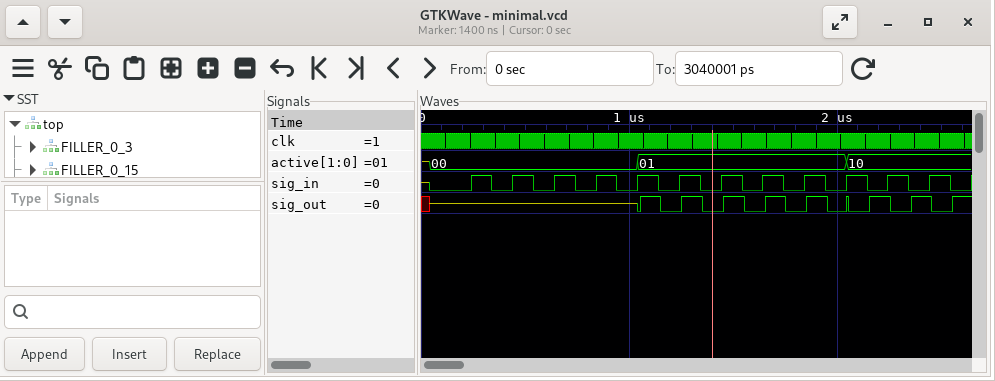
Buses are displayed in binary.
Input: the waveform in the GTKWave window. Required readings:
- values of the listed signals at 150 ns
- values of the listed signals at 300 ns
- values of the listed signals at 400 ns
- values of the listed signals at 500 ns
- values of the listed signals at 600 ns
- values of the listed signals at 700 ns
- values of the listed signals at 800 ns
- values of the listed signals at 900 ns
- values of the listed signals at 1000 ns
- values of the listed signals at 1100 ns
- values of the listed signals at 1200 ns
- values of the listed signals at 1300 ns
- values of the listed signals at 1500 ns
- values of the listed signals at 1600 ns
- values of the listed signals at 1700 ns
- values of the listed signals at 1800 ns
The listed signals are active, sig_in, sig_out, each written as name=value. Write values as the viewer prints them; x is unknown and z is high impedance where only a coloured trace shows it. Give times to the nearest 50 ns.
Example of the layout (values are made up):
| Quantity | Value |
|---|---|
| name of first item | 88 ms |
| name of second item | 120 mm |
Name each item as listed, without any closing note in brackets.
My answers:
| Quantity | Value |
|---|---|
| values of the listed signals at 150 ns | active=00, sig_in=0, sig_out=z |
| values of the listed signals at 300 ns | active=00, sig_in=1, sig_out=z |
| values of the listed signals at 400 ns | active=00, sig_in=0, sig_out=z |
| values of the listed signals at 500 ns | active=00, sig_in=1, sig_out=z |
| values of the listed signals at 600 ns | active=00, sig_in=0, sig_out=z |
| values of the listed signals at 700 ns | active=00, sig_in=1, sig_out=z |
| values of the listed signals at 800 ns | active=00, sig_in=0, sig_out=z |
| values of the listed signals at 900 ns | active=00, sig_in=1, sig_out=z |
| values of the listed signals at 1000 ns | active=00, sig_in=0, sig_out=z |
| values of the listed signals at 1100 ns | active=01, sig_in=1, sig_out=1 |
| values of the listed signals at 1200 ns | active=01, sig_in=0, sig_out=0 |
| values of the listed signals at 1300 ns | active=01, sig_in=1, sig_out=1 |
| values of the listed signals at 1500 ns | active=01, sig_in=1, sig_out=1 |
| values of the listed signals at 1600 ns | active=01, sig_in=0, sig_out=0 |
| values of the listed signals at 1700 ns | active=01, sig_in=1, sig_out=1 |
| values of the listed signals at 1800 ns | active=01, sig_in=0, sig_out=0 |
